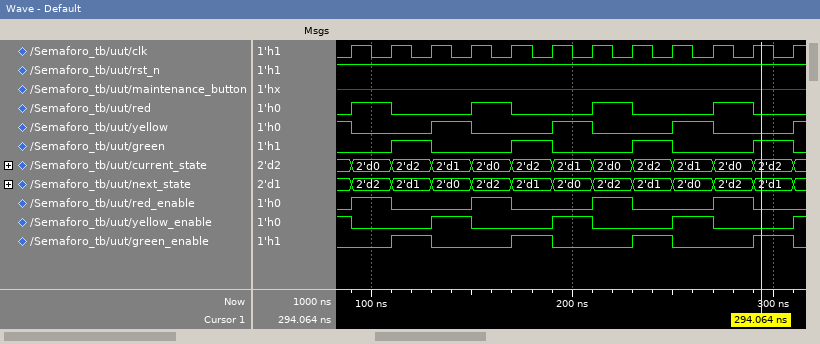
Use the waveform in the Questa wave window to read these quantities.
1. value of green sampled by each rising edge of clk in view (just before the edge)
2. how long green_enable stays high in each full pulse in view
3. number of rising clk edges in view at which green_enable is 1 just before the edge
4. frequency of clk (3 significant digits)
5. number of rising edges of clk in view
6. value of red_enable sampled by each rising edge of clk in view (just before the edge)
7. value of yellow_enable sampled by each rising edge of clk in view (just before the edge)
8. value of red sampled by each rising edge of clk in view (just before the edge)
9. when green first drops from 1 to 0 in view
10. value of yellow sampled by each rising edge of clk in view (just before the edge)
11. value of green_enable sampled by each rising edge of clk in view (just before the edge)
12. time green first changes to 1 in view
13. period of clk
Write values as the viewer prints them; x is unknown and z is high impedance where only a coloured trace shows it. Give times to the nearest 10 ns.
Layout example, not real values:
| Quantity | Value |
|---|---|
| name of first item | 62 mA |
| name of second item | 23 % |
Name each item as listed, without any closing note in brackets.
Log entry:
| Quantity | Value |
|---|---|
| value of green sampled by each rising edge of clk in view | 0 0 1 0 0 1 0 0 1 0 0 1 |
| how long green_enable stays high in each full pulse in view | 20 ns, 20 ns, 20 ns, 20 ns |
| number of rising clk edges in view at which green_enable is 1 just before the edge | 4 |
| frequency of clk | 50.0 MHz |
| number of rising edges of clk in view | 12 |
| value of red_enable sampled by each rising edge of clk in view | 0 1 0 0 1 0 0 1 0 0 1 0 |
| value of yellow_enable sampled by each rising edge of clk in view | 1 0 0 1 0 0 1 0 0 1 0 0 |
| value of red sampled by each rising edge of clk in view | 0 1 0 0 1 0 0 1 0 0 1 0 |
| when green first drops from 1 to 0 in view | 130 ns |
| value of yellow sampled by each rising edge of clk in view | 1 0 0 1 0 0 1 0 0 1 0 0 |
| value of green_enable sampled by each rising edge of clk in view | 0 0 1 0 0 1 0 0 1 0 0 1 |
| time green first changes to 1 in view | 110 ns |
| period of clk | 20 ns |
